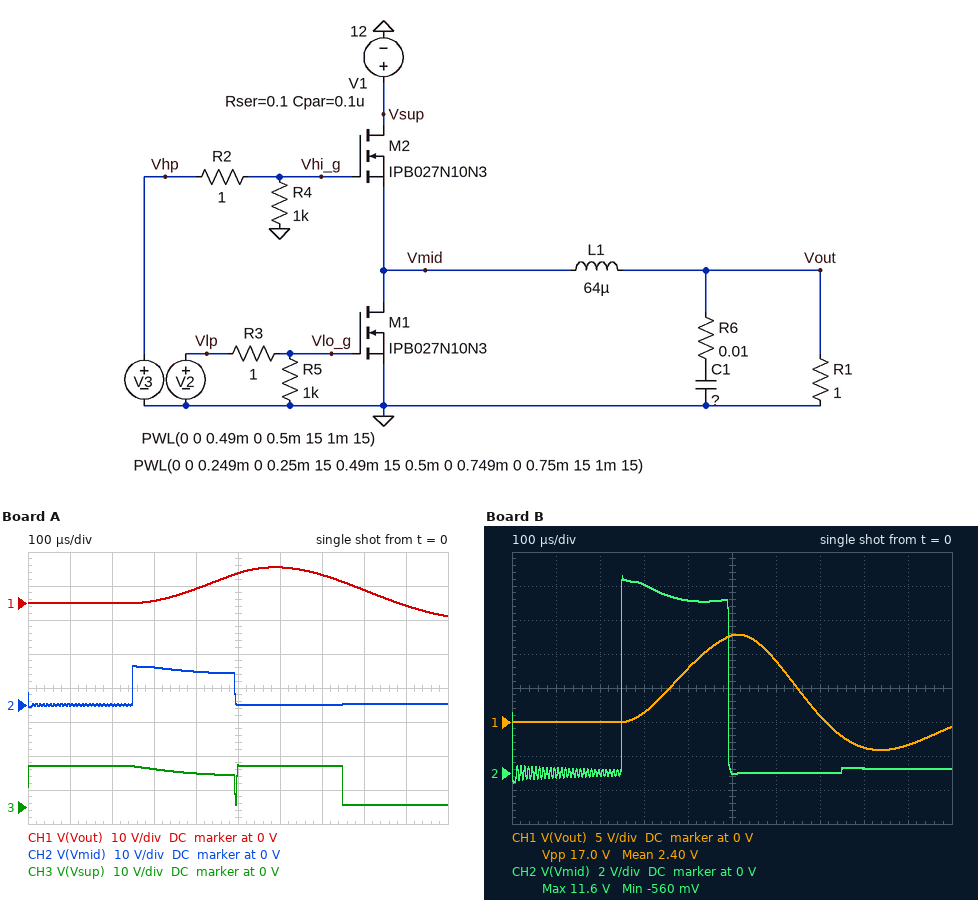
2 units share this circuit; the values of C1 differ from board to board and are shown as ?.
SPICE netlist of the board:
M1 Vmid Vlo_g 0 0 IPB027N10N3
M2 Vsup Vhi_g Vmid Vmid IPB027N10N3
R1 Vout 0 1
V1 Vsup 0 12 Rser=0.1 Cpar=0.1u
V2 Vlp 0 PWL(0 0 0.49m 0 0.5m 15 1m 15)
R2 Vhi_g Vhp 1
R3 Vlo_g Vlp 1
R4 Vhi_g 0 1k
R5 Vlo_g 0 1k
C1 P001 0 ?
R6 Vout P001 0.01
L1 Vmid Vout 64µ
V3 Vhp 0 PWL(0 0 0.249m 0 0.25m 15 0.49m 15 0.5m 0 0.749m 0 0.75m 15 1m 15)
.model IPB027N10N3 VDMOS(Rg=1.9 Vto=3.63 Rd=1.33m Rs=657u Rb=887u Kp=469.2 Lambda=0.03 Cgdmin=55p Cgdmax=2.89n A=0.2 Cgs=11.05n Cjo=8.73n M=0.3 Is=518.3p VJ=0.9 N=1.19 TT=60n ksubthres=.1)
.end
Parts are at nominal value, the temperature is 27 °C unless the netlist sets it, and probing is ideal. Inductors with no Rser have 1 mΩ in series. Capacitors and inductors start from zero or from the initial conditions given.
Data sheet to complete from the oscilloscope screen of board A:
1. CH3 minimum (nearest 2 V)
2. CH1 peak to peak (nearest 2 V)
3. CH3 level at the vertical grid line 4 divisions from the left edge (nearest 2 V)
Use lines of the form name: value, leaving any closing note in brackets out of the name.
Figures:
CH3 minimum: 0 V
CH1 peak to peak: 14 V
CH3 level at the vertical grid line 4 divisions from the left edge: 10 V
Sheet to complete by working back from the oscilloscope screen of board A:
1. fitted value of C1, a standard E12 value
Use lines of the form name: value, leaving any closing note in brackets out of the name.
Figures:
fitted value of C1, a standard E12 value: 390 µF
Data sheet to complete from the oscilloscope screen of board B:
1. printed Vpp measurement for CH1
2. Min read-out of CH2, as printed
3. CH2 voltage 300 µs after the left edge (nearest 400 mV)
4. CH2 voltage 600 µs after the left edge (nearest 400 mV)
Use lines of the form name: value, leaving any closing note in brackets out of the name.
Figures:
printed Vpp measurement for CH1: 17.0 V
Min read-out of CH2, as printed: -560 mV
CH2 voltage 300 µs after the left edge: 11.2 V
CH2 voltage 600 µs after the left edge: 0 V
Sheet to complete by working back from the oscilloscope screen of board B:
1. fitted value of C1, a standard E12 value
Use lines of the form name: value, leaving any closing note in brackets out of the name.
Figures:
fitted value of C1, a standard E12 value: 150 µF
